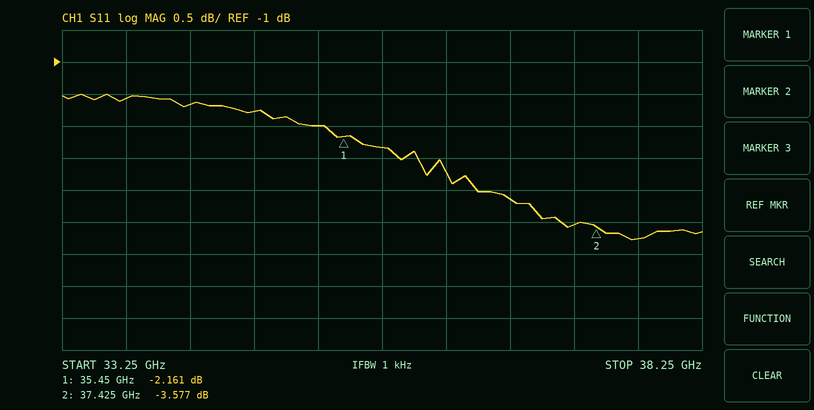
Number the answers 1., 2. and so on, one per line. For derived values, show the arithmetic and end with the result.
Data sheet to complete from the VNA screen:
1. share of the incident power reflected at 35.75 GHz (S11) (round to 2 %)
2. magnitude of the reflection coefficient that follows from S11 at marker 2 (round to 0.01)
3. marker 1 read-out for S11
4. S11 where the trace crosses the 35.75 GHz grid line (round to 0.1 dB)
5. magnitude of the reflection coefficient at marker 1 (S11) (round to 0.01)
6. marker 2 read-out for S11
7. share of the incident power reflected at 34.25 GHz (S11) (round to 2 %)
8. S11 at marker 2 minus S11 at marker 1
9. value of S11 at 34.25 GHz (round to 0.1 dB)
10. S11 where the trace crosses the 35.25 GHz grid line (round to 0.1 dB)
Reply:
1. 10^(-2.3/10) ≈ 58.9 %, so 58 % to the nearest 2 %
2. 10^(-3.577/20) ≈ 0.66
3. -2.161 dB
4. -2.3 dB
5. 10^(-2.161/20) ≈ 0.78
6. -3.577 dB
7. 10^(-1.7/10) ≈ 68 %
8. -3.577 − (-2.161) = -1.416 dB
9. -1.7 dB
10. -2.0 dB
